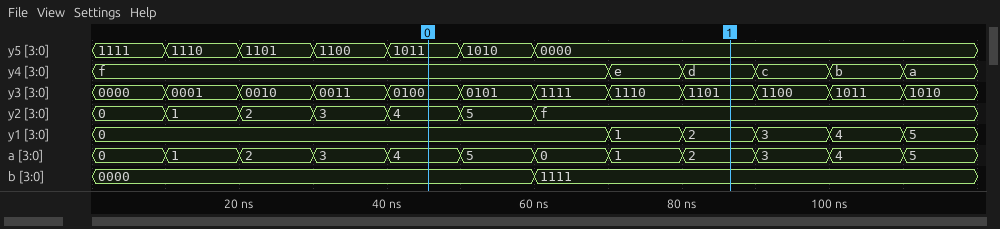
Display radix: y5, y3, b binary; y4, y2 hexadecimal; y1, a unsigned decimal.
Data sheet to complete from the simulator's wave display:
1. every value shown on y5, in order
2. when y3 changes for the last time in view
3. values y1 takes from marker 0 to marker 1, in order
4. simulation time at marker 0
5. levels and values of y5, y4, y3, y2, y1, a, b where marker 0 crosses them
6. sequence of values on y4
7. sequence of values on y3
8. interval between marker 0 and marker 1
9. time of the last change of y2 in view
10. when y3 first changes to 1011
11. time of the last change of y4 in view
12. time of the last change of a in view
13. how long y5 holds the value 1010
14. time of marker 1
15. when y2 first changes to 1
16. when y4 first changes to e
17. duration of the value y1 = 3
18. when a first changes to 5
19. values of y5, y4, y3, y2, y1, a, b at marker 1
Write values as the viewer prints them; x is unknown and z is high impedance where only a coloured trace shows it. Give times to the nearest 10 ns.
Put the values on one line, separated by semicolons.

1111, 1110, 1101, 1100, 1011, 1010, 0000; 110 ns; 0, 1, 2; 50 ns; y5=1011, y4=f, y3=0100, y2=4, y1=0, a=4, b=0000; f, e, d, c, b, a; 0000, 0001, 0010, 0011, 0100, 0101, 1111, 1110, 1101, 1100, 1011, 1010; 40 ns; 60 ns; 100 ns; 110 ns; 110 ns; 10 ns; 90 ns; 10 ns; 70 ns; 10 ns; 50 ns; y5=0000, y4=d, y3=1101, y2=f, y1=2, a=2, b=1111
